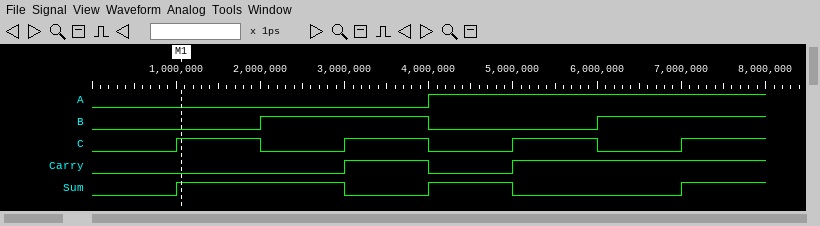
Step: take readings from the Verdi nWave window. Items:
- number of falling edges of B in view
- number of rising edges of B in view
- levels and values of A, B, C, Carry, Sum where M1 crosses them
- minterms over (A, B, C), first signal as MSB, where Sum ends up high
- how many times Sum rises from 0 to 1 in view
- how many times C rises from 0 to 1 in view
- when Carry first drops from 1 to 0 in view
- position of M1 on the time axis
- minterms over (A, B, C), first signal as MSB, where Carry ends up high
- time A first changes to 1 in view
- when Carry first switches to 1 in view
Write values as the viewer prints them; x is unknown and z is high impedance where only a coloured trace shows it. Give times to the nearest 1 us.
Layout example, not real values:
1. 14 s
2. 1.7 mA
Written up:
1. 1
2. 2
3. A=0, B=0, C=1, Carry=0, Sum=1
4. 1, 2, 4, 7
5. 3
6. 4
7. 4 us
8. 1 us
9. 3, 5, 6, 7
10. 4 us
11. 3 us
